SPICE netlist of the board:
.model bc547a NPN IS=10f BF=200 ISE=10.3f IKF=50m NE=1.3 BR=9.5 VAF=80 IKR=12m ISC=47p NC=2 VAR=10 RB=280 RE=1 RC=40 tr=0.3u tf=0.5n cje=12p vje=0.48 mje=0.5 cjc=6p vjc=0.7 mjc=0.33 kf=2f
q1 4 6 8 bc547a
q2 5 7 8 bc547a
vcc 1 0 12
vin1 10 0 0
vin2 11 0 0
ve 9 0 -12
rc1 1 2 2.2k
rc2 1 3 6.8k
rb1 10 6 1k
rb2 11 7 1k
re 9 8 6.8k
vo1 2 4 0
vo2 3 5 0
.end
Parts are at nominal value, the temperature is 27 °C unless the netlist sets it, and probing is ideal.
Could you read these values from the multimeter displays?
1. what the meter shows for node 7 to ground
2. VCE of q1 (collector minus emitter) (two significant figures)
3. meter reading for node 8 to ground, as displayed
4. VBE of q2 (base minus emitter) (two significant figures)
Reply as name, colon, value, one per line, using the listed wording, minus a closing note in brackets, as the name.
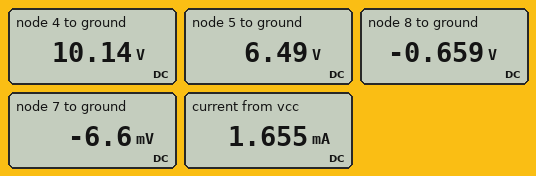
what the meter shows for node 7 to ground: -6.6 mV
VCE of q1 (collector minus emitter): 11 V
meter reading for node 8 to ground, as displayed: -0.659 V
VBE of q2 (base minus emitter): 650 mV
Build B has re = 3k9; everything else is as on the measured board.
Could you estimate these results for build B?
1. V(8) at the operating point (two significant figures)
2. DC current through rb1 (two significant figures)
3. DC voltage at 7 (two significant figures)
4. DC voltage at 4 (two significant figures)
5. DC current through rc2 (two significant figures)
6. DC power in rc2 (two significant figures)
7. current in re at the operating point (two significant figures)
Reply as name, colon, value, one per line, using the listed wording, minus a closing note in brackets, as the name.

V(8) at the operating point: -680 mV
DC current through rb1: 11 µA
DC voltage at 7: -11 mV
DC voltage at 4: 8.7 V
DC current through rc2: 1.4 mA
DC power in rc2: 13 mW
current in re at the operating point: 2.9 mA
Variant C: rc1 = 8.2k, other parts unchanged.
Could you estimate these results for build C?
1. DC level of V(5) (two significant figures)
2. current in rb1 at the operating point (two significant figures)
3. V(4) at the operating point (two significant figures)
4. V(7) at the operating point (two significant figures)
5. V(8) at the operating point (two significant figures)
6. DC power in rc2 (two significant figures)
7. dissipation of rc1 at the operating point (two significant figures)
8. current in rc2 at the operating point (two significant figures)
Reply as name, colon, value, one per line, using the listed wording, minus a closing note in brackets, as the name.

DC level of V(5): 6.3 V
current in rb1 at the operating point: 6.8 µA
V(4) at the operating point: 5.3 V
V(7) at the operating point: -6.8 mV
V(8) at the operating point: -660 mV
DC power in rc2: 4.7 mW
dissipation of rc1 at the operating point: 5.5 mW
current in rc2 at the operating point: 830 µA
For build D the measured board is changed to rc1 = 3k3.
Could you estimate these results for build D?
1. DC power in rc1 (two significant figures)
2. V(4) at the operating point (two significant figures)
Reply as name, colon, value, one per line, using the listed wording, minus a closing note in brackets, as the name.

DC power in rc1: 2.3 mW
V(4) at the operating point: 9.2 V
